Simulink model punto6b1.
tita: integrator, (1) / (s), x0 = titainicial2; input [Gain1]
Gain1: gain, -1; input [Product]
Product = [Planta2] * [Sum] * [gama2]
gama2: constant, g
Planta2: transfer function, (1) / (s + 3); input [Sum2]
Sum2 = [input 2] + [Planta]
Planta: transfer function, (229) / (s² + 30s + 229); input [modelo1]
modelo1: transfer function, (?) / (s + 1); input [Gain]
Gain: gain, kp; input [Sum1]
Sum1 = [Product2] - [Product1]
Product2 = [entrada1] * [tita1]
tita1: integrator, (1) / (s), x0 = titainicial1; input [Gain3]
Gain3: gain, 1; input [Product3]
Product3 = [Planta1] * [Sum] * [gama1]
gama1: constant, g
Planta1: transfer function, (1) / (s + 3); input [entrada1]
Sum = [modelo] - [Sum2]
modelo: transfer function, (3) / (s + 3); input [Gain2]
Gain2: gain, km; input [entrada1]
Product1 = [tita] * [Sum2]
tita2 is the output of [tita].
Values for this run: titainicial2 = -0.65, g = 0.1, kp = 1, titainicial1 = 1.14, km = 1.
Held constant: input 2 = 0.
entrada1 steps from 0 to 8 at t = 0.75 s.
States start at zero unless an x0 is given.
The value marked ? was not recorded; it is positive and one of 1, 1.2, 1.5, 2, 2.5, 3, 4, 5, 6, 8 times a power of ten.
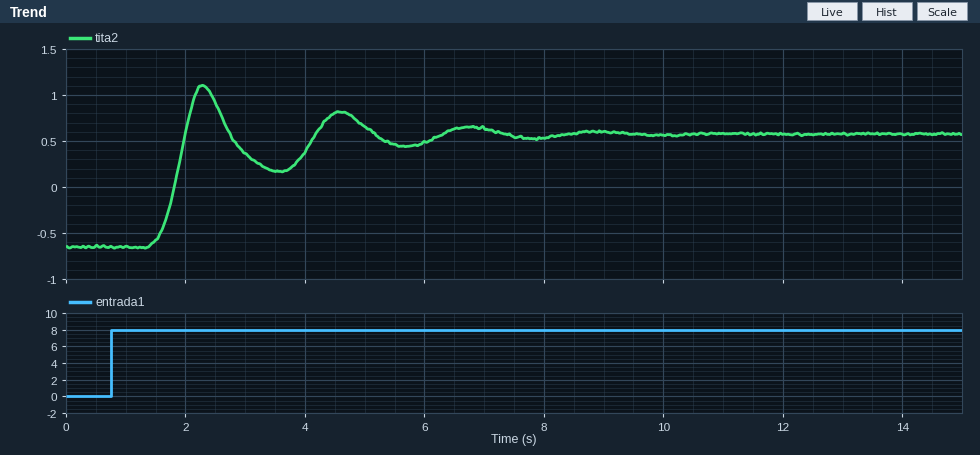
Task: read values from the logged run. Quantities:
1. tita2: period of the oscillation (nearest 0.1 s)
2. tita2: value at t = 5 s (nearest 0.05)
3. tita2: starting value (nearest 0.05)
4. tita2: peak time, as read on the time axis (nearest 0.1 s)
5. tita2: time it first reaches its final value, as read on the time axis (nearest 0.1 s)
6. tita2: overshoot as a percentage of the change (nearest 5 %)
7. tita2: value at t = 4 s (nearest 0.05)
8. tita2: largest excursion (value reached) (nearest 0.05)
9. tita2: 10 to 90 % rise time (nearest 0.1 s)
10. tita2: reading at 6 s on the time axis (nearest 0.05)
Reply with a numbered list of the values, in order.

1. 2.3 s
2. 0.65
3. -0.65
4. 2.3 s
5. 2.0 s
6. 45 %
7. 0.40
8. 1.10
9. 0.4 s
10. 0.50
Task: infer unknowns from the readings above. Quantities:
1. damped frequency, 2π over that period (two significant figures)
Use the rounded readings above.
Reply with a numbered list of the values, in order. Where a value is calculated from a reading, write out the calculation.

1. 2π / 2.3 = 2.7 rad/s
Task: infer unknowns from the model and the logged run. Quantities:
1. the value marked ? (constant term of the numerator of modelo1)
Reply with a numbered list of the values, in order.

1. 2
